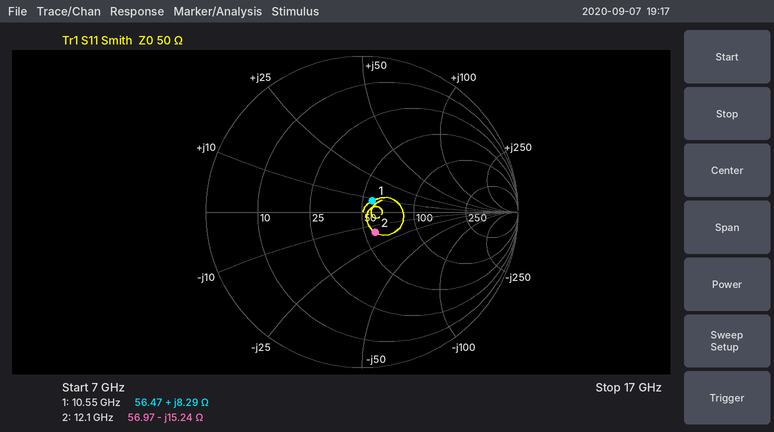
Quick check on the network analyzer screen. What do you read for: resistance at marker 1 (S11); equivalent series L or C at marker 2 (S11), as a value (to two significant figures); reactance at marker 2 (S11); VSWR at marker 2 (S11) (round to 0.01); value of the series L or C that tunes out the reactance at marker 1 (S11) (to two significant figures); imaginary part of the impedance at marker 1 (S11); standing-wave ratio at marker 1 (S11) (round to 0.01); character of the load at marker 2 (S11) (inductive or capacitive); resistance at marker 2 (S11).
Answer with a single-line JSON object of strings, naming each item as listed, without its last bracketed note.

{"resistance at marker 1": "56.47 Ω", "equivalent series L or C at marker 2 (S11), as a value": "860 fF", "reactance at marker 2": "-15.24 Ω", "VSWR at marker 2 (S11)": "1.37", "value of the series L or C that tunes out the reactance at marker 1 (S11)": "1.8 pF", "imaginary part of the impedance at marker 1": "+8.29 Ω", "standing-wave ratio at marker 1 (S11)": "1.22", "character of the load at marker 2 (S11)": "capacitive", "resistance at marker 2": "56.97 Ω"}
